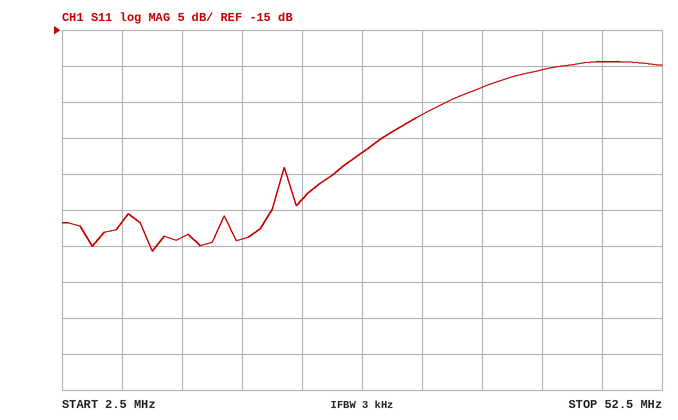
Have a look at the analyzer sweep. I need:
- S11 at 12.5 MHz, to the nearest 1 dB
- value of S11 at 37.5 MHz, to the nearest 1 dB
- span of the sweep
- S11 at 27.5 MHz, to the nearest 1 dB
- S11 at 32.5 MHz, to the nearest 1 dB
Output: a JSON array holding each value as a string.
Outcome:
["-44 dB", "-23 dB", "50 MHz", "-32 dB", "-27 dB"]
